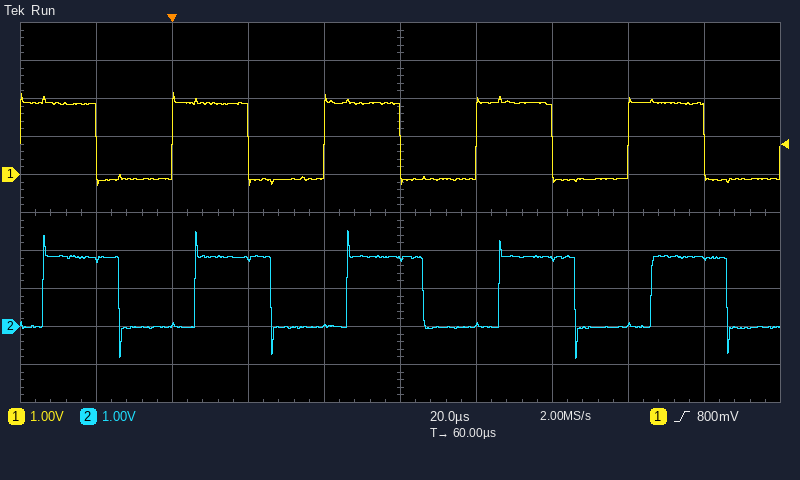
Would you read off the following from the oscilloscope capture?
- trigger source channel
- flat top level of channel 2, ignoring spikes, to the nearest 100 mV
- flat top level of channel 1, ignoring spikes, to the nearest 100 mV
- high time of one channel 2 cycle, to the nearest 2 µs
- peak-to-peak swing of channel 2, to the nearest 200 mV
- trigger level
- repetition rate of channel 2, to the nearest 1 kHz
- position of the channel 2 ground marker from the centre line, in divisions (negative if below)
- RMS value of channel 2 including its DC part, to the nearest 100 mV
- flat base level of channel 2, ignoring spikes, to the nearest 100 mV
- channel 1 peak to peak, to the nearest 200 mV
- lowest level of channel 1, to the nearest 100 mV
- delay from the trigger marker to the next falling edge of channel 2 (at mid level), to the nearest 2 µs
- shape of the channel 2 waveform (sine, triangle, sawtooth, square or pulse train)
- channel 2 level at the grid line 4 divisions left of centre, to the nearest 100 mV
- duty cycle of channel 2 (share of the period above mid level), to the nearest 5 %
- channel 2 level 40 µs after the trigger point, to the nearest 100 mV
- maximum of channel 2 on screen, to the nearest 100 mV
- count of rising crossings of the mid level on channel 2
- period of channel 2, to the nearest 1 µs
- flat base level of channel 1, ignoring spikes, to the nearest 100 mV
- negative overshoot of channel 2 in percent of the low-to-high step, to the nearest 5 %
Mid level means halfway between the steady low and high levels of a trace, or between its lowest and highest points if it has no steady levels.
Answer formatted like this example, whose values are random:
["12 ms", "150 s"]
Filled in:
["channel 1", "1.8 V", "1.9 V", "20 µs", "3.4 V", "800 mV", "25 kHz", "-3.0 div", "1.3 V", "0.0 V", "2.4 V", "-300 mV", "26 µs", "square", "1.8 V", "50 %", "0.0 V", "2.5 V", "5", "40 µs", "-100 mV", "45 %"]
